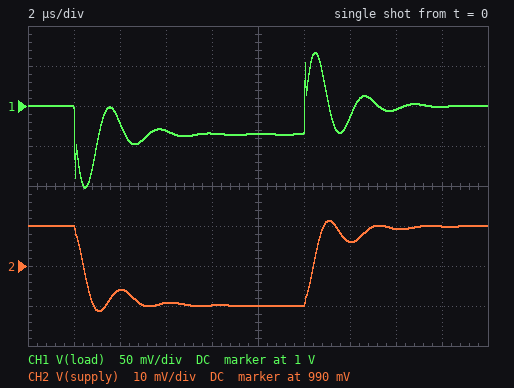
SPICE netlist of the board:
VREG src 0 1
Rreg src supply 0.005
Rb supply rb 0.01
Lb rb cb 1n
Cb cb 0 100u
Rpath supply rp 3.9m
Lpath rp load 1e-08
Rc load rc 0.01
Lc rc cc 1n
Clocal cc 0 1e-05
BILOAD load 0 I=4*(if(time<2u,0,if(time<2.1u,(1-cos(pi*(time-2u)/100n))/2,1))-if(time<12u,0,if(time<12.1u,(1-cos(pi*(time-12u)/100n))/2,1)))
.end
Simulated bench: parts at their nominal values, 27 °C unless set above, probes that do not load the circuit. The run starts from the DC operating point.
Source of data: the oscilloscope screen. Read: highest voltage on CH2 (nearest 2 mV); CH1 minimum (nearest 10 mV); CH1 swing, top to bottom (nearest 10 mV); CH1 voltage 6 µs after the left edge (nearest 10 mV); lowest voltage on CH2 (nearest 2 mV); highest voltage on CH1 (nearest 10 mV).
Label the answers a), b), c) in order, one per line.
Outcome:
a) 1.002 V
b) 900 mV
c) 170 mV
d) 970 mV
e) 978 mV
f) 1.07 V
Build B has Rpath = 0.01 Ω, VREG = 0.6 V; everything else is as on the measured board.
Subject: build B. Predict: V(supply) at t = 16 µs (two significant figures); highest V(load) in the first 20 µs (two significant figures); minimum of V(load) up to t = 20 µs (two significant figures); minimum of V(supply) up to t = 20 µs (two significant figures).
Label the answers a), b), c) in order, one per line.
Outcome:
a) 600 mV
b) 650 mV
c) 490 mV
d) 580 mV
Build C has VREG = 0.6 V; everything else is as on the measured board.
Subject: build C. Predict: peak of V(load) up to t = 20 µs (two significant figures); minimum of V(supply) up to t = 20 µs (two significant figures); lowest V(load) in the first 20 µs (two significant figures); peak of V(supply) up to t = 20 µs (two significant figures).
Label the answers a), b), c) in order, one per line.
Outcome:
a) 670 mV
b) 580 mV
c) 500 mV
d) 600 mV
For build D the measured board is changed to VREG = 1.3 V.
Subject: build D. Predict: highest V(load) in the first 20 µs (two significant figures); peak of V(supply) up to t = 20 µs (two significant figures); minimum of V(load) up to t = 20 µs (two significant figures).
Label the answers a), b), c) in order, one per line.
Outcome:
a) 1.4 V
b) 1.3 V
c) 1.2 V
